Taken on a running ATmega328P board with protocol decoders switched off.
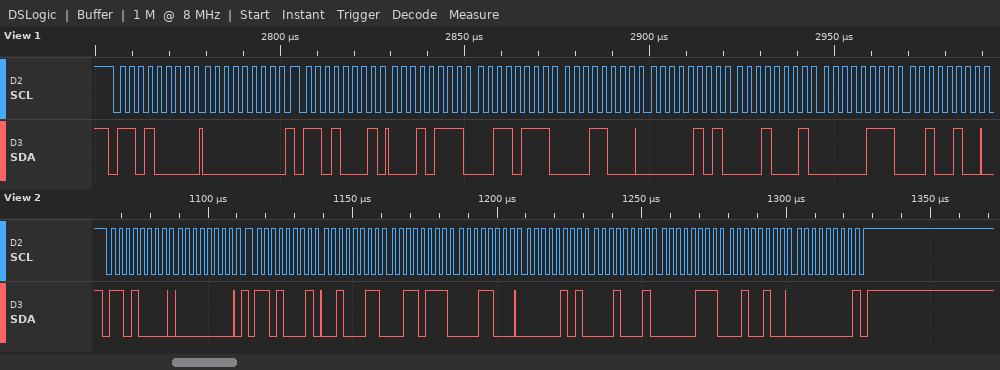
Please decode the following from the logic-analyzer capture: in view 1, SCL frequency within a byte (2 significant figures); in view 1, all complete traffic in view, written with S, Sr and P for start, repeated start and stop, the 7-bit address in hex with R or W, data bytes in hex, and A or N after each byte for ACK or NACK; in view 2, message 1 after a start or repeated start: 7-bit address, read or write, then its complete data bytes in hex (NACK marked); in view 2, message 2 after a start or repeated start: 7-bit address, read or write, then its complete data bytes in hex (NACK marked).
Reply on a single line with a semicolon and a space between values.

400 kHz; S 68W A 00 A Sr 68R A 17 A 37 A 18 A 05 A 11 A 07 A 24 A; 0x68 write: 00; 0x68 read: 23 37 18 05 11 07 24 00 NACK
